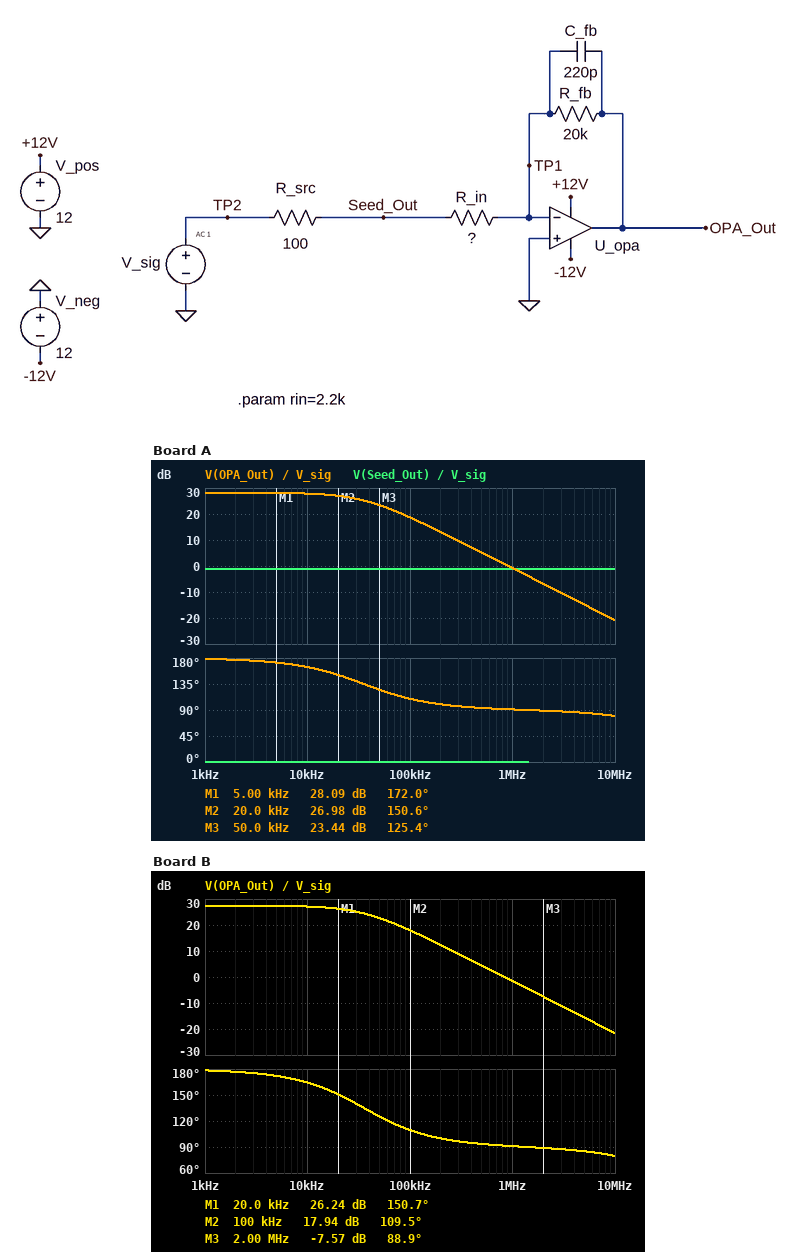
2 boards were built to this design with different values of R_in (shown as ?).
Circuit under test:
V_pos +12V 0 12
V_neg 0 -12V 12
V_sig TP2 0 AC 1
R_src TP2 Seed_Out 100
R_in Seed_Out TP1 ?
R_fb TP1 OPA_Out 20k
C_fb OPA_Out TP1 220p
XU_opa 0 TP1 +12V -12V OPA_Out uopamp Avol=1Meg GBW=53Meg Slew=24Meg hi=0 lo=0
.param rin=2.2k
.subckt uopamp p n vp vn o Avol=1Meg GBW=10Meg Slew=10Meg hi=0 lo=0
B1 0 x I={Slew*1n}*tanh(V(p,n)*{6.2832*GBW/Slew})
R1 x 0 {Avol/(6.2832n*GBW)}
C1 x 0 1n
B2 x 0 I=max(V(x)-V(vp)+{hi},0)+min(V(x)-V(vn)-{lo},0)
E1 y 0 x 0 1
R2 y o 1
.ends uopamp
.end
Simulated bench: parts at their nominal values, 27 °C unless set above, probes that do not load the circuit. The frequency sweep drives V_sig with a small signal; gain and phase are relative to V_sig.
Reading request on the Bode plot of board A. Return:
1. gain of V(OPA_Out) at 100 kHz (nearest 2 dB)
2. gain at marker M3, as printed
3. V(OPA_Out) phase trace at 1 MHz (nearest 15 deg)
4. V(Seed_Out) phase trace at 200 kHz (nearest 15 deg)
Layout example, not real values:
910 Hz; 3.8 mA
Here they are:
18 dB; 23.44 dB; 90 deg; 0 deg
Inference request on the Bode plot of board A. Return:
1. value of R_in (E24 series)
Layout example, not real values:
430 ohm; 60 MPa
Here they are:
680 Ω
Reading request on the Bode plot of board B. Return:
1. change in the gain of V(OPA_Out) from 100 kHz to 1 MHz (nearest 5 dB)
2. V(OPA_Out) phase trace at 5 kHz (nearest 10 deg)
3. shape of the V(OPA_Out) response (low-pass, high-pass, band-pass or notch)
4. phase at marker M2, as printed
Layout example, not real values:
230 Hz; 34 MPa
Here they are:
-20 dB; 170 deg; low-pass; 109.5 deg
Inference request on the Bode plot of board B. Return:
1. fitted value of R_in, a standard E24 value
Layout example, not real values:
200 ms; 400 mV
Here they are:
750 Ω
